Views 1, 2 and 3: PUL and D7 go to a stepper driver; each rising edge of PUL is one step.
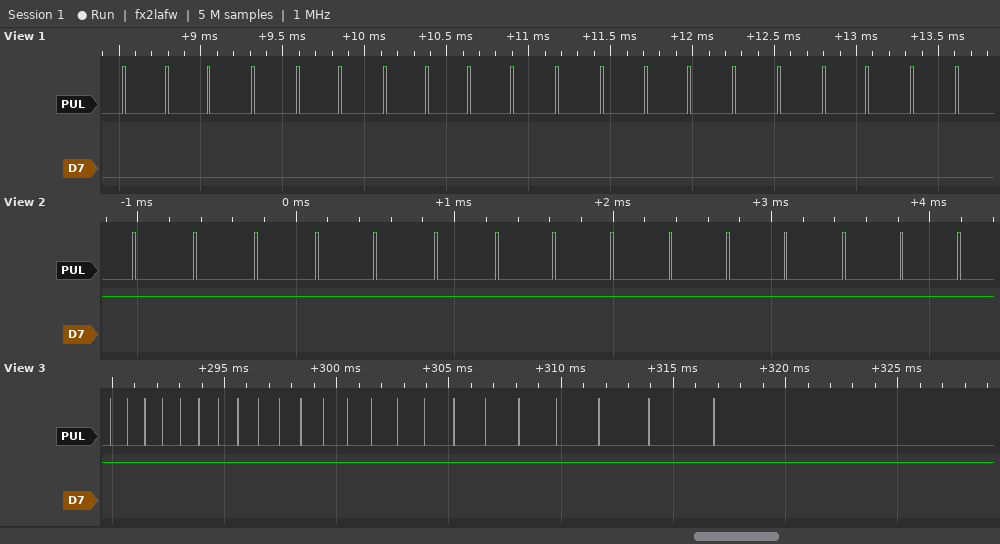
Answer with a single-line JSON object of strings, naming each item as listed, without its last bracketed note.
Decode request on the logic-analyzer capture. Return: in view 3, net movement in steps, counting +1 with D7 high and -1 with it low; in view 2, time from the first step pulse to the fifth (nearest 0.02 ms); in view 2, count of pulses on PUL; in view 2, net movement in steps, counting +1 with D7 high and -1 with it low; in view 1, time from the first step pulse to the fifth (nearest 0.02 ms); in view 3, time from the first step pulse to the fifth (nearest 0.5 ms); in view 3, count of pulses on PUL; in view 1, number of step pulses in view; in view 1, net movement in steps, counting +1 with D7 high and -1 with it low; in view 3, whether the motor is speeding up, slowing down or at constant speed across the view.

{"in view 3, net movement in steps, counting +1 with D7 high and -1 with it low": "+23", "in view 2, time from the first step pulse to the fifth": "1.52 ms", "in view 2, count of pulses on PUL": "15", "in view 2, net movement in steps, counting +1 with D7 high and -1 with it low": "+15", "in view 1, time from the first step pulse to the fifth": "1.06 ms", "in view 3, time from the first step pulse to the fifth": "3.0 ms", "in view 3, count of pulses on PUL": "23", "in view 1, number of step pulses in view": "20", "in view 1, net movement in steps, counting +1 with D7 high and -1 with it low": "-20", "in view 3, whether the motor is speeding up, slowing down or at constant speed across the view": "slowing down"}
